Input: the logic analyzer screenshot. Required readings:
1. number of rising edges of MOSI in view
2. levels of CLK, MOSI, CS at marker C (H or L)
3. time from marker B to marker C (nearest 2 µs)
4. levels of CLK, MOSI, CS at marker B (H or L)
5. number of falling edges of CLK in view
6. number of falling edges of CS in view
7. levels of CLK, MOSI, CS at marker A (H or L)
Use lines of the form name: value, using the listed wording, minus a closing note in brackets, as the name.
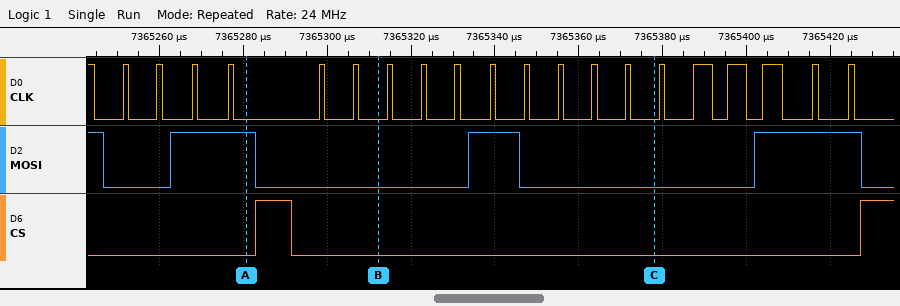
number of rising edges of MOSI in view: 3
levels of CLK, MOSI, CS at marker C: CLK=L, MOSI=L, CS=L
time from marker B to marker C: 66 µs
levels of CLK, MOSI, CS at marker B: CLK=L, MOSI=L, CS=L
number of falling edges of CLK in view: 21
number of falling edges of CS in view: 1
levels of CLK, MOSI, CS at marker A: CLK=L, MOSI=H, CS=L
